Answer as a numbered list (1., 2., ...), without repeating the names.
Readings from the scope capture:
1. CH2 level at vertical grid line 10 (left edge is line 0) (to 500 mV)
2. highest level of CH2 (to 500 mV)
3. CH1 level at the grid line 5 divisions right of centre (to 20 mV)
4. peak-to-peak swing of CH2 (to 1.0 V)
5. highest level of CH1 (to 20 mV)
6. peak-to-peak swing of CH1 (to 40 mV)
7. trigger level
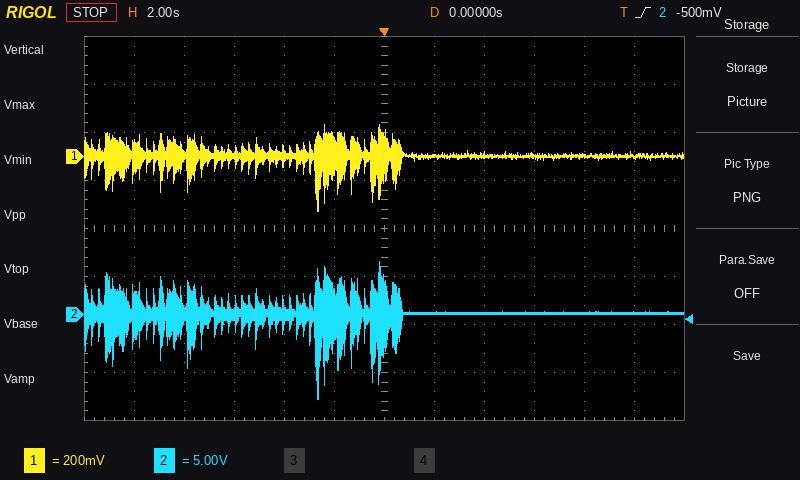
1. 0.0 V
2. 5.5 V
3. 0 mV
4. 14.0 V
5. 140 mV
6. 360 mV
7. -500 mV
